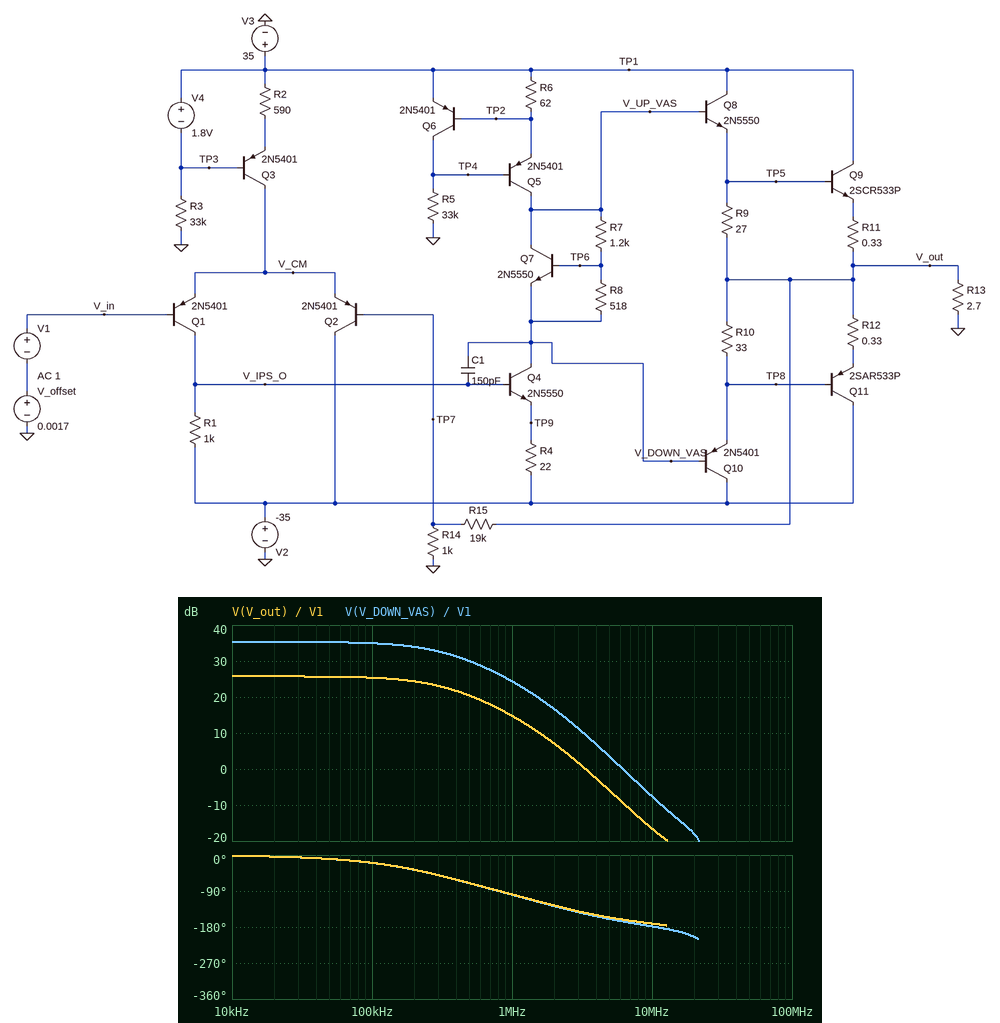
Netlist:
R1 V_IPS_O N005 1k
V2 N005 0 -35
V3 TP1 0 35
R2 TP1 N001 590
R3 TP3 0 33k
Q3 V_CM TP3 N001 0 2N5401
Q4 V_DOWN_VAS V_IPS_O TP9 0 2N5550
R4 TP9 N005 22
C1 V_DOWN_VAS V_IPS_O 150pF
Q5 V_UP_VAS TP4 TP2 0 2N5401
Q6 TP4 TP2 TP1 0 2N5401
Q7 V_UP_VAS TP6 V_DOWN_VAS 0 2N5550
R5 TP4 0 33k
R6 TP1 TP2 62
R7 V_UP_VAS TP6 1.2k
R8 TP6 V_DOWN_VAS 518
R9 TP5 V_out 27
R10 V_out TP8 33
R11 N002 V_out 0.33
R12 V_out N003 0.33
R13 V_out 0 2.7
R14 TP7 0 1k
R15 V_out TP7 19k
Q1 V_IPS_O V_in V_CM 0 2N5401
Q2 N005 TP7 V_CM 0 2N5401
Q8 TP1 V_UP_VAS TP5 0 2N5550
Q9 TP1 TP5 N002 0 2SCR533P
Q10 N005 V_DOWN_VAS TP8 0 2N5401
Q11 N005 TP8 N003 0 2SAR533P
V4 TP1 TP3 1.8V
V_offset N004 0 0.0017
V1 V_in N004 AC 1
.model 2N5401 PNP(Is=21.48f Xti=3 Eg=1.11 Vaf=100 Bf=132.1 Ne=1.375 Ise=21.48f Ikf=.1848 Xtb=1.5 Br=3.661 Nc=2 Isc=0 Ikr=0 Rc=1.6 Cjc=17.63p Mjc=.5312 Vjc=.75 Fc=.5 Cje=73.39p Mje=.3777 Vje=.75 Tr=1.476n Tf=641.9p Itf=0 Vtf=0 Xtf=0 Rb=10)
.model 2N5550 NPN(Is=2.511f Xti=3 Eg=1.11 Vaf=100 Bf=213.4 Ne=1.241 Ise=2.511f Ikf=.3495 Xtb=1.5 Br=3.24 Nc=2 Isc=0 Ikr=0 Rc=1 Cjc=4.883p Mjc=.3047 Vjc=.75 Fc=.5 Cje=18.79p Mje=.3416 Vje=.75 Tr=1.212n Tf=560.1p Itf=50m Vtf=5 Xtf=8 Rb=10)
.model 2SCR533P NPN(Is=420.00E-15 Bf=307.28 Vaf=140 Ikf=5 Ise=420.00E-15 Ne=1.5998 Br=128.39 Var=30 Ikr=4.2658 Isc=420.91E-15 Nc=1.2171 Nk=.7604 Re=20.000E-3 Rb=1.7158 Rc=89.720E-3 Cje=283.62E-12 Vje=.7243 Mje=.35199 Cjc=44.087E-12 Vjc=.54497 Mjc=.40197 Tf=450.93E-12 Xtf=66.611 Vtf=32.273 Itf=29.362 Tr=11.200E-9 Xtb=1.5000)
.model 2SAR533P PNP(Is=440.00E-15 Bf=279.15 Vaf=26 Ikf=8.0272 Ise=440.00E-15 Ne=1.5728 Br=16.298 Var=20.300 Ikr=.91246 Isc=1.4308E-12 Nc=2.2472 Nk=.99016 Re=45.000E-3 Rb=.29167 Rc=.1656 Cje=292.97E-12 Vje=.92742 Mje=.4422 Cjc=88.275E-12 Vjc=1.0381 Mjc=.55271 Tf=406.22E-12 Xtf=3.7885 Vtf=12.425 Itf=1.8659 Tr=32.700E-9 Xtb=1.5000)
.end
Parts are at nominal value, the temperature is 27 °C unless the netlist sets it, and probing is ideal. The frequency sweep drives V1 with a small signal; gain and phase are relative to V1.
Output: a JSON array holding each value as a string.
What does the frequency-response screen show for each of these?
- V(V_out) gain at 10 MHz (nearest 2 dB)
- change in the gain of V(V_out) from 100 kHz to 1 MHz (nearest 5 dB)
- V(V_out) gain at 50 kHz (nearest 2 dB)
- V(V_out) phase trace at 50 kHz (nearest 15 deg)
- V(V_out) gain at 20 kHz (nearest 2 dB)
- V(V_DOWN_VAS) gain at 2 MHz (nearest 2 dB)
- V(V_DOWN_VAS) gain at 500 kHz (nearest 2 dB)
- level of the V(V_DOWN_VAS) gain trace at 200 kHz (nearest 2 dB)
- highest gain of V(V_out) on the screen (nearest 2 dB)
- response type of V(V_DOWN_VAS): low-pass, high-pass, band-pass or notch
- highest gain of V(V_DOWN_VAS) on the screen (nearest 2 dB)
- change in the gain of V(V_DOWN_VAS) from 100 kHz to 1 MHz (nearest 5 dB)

["-16 dB", "-10 dB", "26 dB", "-15 deg", "26 dB", "16 dB", "30 dB", "34 dB", "26 dB", "low-pass", "36 dB", "-10 dB"]
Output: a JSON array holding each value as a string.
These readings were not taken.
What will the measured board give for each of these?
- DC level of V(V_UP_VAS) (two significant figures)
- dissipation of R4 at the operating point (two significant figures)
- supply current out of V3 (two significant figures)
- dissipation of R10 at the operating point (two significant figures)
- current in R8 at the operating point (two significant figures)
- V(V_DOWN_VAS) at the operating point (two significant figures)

["1.3 V", "2.3 mW", "34 mA", "9.7 mW", "1.4 mA", "-1.3 V"]
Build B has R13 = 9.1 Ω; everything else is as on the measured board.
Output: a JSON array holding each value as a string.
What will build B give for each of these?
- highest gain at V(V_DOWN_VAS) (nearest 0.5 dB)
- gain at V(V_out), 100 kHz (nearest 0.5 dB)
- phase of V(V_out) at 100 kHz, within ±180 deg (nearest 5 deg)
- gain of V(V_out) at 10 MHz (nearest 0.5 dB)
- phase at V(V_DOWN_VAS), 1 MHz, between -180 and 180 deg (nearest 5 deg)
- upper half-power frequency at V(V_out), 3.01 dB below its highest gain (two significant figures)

["30.0 dB", "26.0 dB", "-10 deg", "-11.5 dB", "-85 deg", "680 kHz"]
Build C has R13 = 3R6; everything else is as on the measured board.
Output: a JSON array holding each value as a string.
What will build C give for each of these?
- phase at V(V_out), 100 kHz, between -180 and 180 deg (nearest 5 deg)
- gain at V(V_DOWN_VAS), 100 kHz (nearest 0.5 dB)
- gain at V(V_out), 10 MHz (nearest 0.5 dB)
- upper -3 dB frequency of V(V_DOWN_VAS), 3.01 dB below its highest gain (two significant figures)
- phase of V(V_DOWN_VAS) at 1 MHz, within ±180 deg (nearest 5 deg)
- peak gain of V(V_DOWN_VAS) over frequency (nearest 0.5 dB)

["-15 deg", "33.5 dB", "-15.0 dB", "400 kHz", "-95 deg", "34.0 dB"]
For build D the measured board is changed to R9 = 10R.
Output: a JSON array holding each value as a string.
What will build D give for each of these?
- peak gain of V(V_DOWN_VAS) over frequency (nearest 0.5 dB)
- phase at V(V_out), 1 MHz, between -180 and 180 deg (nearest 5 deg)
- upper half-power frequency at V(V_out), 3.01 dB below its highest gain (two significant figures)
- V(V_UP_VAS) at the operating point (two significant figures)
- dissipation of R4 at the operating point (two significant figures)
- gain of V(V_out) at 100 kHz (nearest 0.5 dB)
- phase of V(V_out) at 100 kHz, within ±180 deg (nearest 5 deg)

["29.0 dB", "-80 deg", "770 kHz", "1.2 V", "2.2 mW", "26.0 dB", "-10 deg"]
